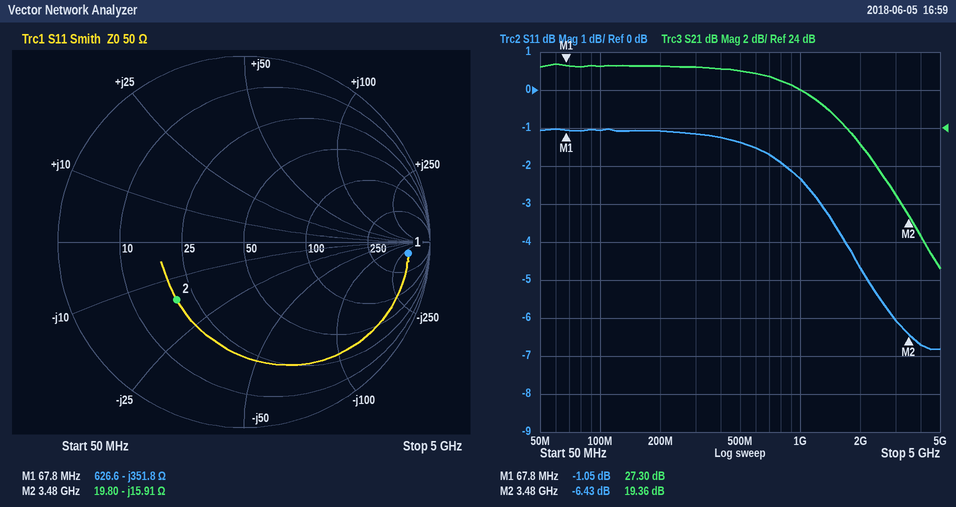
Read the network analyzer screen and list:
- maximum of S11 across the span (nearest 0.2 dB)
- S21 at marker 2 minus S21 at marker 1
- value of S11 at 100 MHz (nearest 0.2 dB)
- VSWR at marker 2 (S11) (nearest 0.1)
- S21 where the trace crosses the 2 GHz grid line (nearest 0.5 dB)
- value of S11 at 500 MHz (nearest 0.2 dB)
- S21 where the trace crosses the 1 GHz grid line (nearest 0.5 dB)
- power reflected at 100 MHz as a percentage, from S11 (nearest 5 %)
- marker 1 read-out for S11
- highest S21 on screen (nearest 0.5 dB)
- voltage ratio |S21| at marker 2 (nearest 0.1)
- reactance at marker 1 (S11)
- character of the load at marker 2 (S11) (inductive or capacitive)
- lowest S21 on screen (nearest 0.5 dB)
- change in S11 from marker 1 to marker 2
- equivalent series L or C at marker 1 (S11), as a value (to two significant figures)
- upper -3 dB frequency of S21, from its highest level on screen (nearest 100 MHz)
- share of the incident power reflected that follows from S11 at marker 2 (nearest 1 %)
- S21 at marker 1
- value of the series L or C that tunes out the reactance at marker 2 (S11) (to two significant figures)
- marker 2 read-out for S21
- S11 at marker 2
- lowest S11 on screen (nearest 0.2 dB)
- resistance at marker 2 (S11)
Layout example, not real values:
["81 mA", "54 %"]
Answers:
["-1.0 dB", "-7.94 dB", "-1.0 dB", "2.8", "23.0 dB", "-1.4 dB", "26.0 dB", "80 %", "-1.05 dB", "27.5 dB", "9.3", "-351.8 Ω", "capacitive", "16.5 dB", "-5.38 dB", "6.7 pF", "1.6 GHz", "23 %", "27.30 dB", "730 pH", "19.36 dB", "-6.43 dB", "-6.8 dB", "19.80 Ω"]
